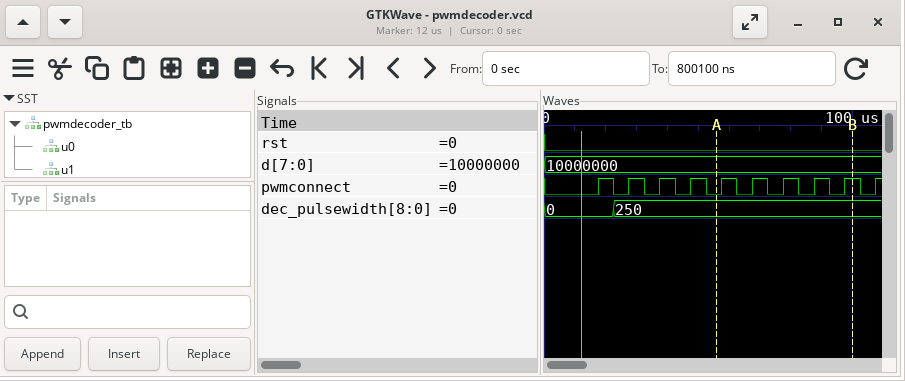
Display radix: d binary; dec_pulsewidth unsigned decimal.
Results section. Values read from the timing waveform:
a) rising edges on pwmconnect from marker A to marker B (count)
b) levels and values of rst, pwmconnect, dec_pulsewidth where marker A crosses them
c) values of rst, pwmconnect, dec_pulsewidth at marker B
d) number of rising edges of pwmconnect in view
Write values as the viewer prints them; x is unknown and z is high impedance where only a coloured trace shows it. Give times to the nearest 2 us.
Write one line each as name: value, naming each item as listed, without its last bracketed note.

rising edges on pwmconnect from marker A to marker B: 5
levels and values of rst, pwmconnect, dec_pulsewidth where marker A crosses them: rst=0, pwmconnect=0, dec_pulsewidth=250
values of rst, pwmconnect, dec_pulsewidth at marker B: rst=0, pwmconnect=1, dec_pulsewidth=250
number of rising edges of pwmconnect in view: 10
